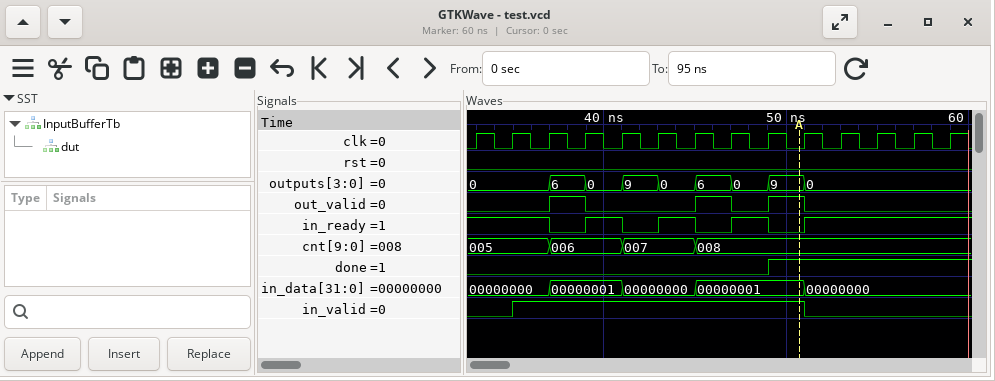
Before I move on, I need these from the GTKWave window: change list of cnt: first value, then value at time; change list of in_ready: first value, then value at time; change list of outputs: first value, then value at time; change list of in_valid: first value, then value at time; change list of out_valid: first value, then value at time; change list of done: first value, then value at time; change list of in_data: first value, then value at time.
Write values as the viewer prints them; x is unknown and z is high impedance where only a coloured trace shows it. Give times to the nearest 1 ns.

005, 006 at 37 ns, 007 at 41 ns, 008 at 45 ns
1, 0 at 37 ns, 1 at 39 ns, 0 at 41 ns, 1 at 43 ns, 0 at 45 ns, 1 at 47 ns, 0 at 49 ns, 1 at 51 ns
0, 6 at 37 ns, 0 at 39 ns, 9 at 41 ns, 0 at 43 ns, 6 at 45 ns, 0 at 47 ns, 9 at 49 ns, 0 at 51 ns
0, 1 at 35 ns, 0 at 51 ns
0, 1 at 37 ns, 0 at 39 ns, 1 at 45 ns, 0 at 47 ns, 1 at 49 ns, 0 at 51 ns
0, 1 at 49 ns
00000000, 00000001 at 37 ns, 00000000 at 41 ns, 00000001 at 45 ns, 00000000 at 51 ns
